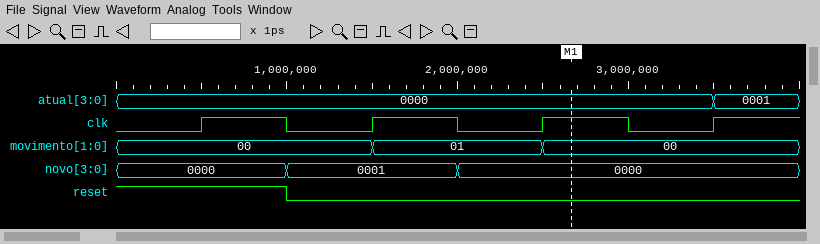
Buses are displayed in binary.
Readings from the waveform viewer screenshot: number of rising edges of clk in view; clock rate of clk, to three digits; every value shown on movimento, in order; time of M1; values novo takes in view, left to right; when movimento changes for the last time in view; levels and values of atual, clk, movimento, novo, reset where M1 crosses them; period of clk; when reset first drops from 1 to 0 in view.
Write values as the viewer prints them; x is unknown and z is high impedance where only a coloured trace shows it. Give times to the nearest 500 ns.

4
1.00 MHz
00, 01, 00
2500 ns
0000, 0001, 0000
2500 ns
atual=0000, clk=1, movimento=00, novo=0000, reset=0
1000 ns
1000 ns
